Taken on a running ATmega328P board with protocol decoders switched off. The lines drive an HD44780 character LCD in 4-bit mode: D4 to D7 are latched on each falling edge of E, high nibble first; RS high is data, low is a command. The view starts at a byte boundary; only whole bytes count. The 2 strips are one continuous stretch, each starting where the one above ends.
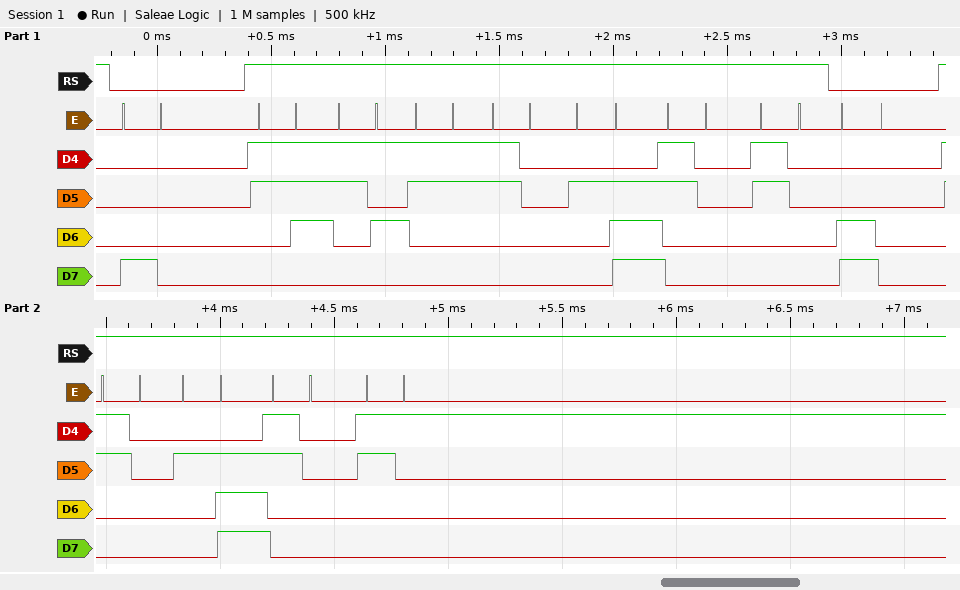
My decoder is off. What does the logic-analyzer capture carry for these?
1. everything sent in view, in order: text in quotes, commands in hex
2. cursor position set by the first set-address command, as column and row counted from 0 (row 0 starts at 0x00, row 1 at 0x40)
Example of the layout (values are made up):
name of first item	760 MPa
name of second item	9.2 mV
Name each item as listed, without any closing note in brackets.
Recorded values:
everything sent in view, in order: text in quotes, commands in hex	0x80 "7530.00" 0xC0 "0.01"
cursor position set by the first set-address command, as column and row counted from 0	column 0, row 0
